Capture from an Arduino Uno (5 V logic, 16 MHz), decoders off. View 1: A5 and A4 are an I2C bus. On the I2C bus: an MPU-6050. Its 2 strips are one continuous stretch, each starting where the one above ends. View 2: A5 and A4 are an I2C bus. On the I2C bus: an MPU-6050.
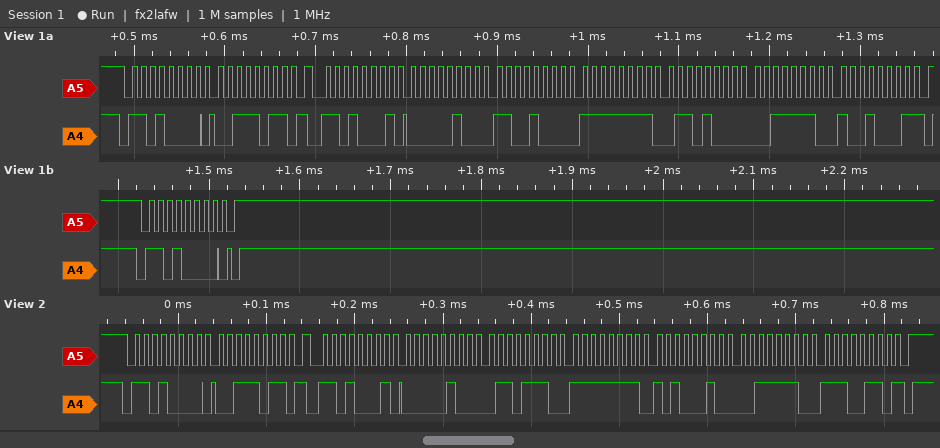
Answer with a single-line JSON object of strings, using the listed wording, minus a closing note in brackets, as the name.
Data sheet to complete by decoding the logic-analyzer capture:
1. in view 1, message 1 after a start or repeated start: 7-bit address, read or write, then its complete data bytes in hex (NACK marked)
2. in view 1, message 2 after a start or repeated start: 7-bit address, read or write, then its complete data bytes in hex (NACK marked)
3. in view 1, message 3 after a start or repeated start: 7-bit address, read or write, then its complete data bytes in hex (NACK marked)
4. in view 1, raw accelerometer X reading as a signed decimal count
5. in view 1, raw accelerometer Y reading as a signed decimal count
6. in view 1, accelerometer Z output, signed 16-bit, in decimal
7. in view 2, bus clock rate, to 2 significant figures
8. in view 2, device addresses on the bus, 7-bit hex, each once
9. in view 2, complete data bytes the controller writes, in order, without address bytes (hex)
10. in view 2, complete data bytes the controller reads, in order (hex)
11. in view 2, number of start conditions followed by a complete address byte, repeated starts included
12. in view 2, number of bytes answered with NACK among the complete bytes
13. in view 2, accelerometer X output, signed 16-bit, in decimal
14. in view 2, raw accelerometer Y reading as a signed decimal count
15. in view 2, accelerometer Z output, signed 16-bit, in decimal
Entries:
{"in view 1, message 1 after a start or repeated start: 7-bit address, read or write, then its complete data bytes in hex": "0x68 write: 3B", "in view 1, message 2 after a start or repeated start: 7-bit address, read or write, then its complete data bytes in hex": "0x68 read: 04 C8 FF 68 3E 91 NACK", "in view 1, message 3 after a start or repeated start: 7-bit address, read or write, then its complete data bytes in hex": "0x68 write", "in view 1, raw accelerometer X reading as a signed decimal count": "1224", "in view 1, raw accelerometer Y reading as a signed decimal count": "-152", "in view 1, accelerometer Z output, signed 16-bit, in decimal": "16017", "in view 2, bus clock rate, to 2 significant figures": "100 kHz", "in view 2, device addresses on the bus, 7-bit hex, each once": "0x68", "in view 2, complete data bytes the controller writes, in order, without address bytes": "3B", "in view 2, complete data bytes the controller reads, in order": "04 6E FF A2 3E E6", "in view 2, number of start conditions followed by a complete address byte, repeated starts included": "2", "in view 2, number of bytes answered with NACK among the complete bytes": "1", "in view 2, accelerometer X output, signed 16-bit, in decimal": "1134", "in view 2, raw accelerometer Y reading as a signed decimal count": "-94", "in view 2, accelerometer Z output, signed 16-bit, in decimal": "16102"}
